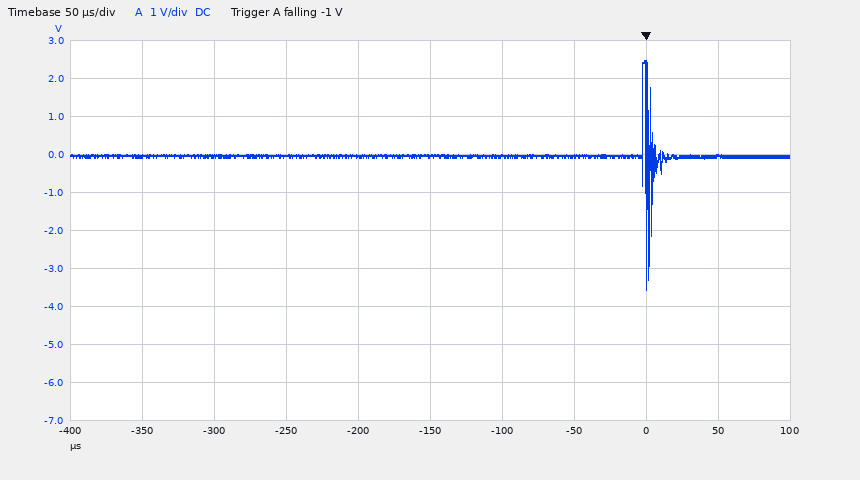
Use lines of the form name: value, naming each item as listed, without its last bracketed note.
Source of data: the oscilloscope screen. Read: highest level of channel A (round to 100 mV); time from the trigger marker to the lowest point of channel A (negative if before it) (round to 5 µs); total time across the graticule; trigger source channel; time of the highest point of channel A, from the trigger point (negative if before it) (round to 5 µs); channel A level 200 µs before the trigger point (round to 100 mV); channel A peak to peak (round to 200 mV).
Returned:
highest level of channel A: 2.5 V
time from the trigger marker to the lowest point of channel A (negative if before it): 0 µs
total time across the graticule: 500 µs
trigger source channel: channel A
time of the highest point of channel A, from the trigger point (negative if before it): 0 µs
channel A level 200 µs before the trigger point: 0.0 V
channel A peak to peak: 6.0 V
